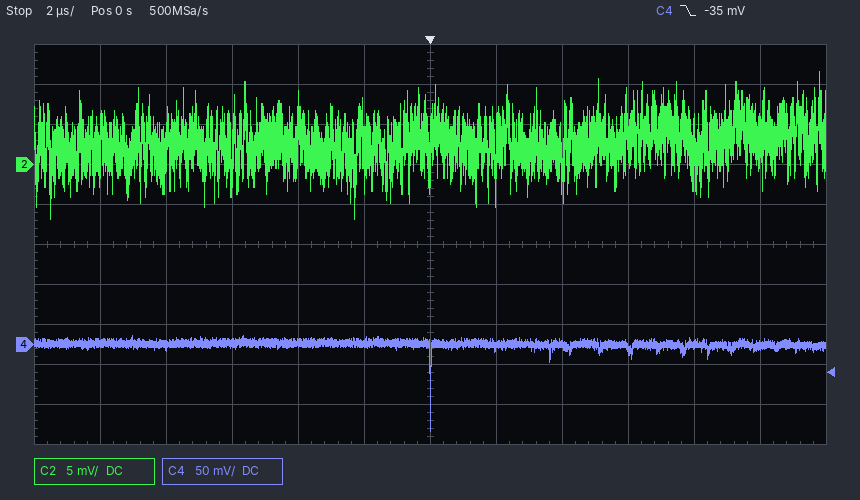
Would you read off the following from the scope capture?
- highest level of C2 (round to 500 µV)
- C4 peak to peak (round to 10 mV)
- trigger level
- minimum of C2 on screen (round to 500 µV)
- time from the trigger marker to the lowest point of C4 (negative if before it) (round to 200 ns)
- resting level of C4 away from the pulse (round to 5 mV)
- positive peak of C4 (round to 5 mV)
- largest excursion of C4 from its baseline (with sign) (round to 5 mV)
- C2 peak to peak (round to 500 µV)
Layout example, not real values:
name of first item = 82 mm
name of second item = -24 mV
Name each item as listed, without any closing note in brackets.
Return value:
highest level of C2 = 11.5 mV
C4 peak to peak = 120 mV
trigger level = -35 mV
minimum of C2 on screen = -7.0 mV
time from the trigger marker to the lowest point of C4 (negative if before it) = 0.0 µs
resting level of C4 away from the pulse = 0 mV
positive peak of C4 = 10 mV
largest excursion of C4 from its baseline (with sign) = -110 mV
C2 peak to peak = 18.5 mV
